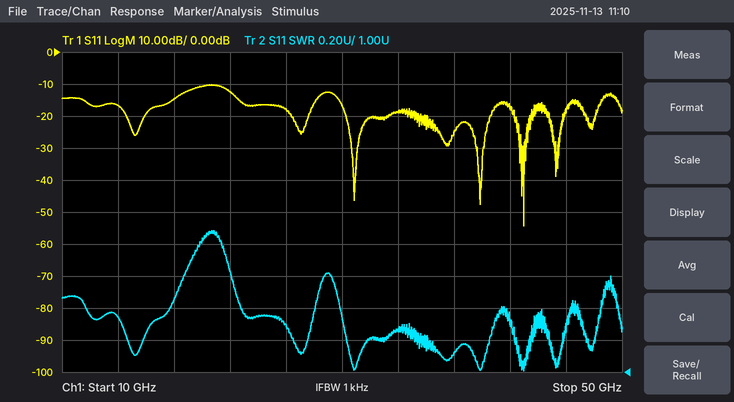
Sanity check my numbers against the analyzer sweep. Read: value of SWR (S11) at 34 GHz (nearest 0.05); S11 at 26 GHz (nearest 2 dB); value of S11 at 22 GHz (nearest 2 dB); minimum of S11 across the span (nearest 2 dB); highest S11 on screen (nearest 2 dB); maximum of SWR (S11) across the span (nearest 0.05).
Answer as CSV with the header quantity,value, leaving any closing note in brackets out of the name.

quantity,value
value of SWR (S11) at 34 GHz,1.25
S11 at 26 GHz,-18 dB
value of S11 at 22 GHz,-12 dB
minimum of S11 across the span,-54 dB
highest S11 on screen,-10 dB
maximum of SWR (S11) across the span,1.90
